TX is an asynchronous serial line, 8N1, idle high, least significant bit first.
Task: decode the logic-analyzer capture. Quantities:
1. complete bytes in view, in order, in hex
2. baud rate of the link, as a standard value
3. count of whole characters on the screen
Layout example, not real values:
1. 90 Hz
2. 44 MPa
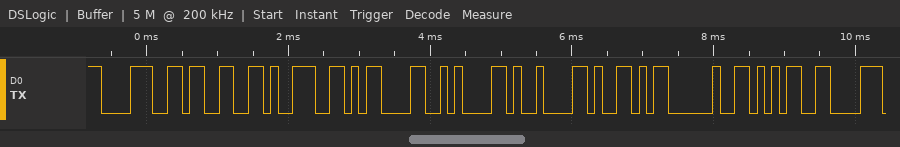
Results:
1. 0x38 0x33 0x39 0x0D 0x0A 0x09 0x59 0x20 0x35
2. 9600 baud
3. 9
